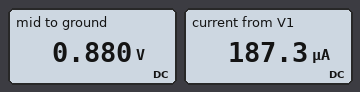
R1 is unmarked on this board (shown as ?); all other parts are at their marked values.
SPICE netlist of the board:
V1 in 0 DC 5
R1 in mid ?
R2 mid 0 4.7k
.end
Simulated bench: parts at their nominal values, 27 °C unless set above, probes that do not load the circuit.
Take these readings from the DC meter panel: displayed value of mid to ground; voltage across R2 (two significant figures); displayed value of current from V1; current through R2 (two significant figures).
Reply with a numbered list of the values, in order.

1. 0.880 V
2. 880 mV
3. 187.3 µA
4. 190 µA
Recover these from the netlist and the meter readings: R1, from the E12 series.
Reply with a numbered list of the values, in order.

1. 22 kΩ
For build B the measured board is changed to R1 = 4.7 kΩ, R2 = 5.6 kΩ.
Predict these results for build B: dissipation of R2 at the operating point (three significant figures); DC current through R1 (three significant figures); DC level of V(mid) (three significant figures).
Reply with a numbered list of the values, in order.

1. 1.32 mW
2. 485 µA
3. 2.72 V
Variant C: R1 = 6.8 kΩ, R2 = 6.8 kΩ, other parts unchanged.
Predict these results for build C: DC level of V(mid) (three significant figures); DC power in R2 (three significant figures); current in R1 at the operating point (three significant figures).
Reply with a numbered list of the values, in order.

1. 2.50 V
2. 919 µW
3. 368 µA
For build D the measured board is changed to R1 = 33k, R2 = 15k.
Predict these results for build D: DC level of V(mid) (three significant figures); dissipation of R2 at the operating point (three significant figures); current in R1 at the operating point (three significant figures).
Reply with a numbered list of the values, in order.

1. 1.56 V
2. 163 µW
3. 104 µA
